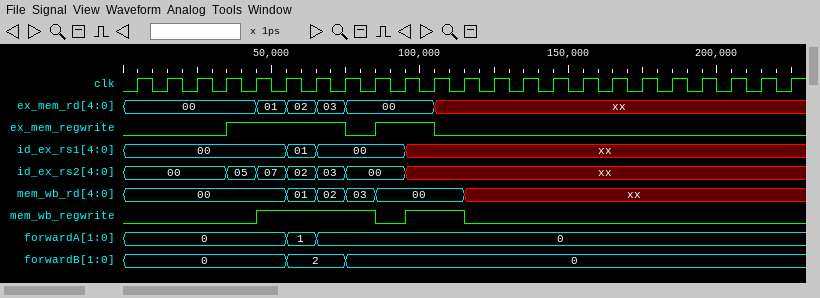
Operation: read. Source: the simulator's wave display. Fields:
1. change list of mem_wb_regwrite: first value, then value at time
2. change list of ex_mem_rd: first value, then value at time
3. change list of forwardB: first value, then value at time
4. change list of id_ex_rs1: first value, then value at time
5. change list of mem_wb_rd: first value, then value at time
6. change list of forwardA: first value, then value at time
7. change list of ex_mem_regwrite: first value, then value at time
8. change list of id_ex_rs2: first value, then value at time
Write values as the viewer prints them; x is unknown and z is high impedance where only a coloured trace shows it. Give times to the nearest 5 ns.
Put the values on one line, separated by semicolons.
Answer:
0, 1 at 45 ns, 0 at 85 ns, 1 at 95 ns, 0 at 115 ns; 00, 01 at 45 ns, 02 at 55 ns, 03 at 65 ns, 00 at 75 ns, xx at 105 ns; 0, 2 at 55 ns, 0 at 75 ns; 00, 01 at 55 ns, 00 at 65 ns, xx at 95 ns; 00, 01 at 55 ns, 02 at 65 ns, 03 at 75 ns, 00 at 85 ns, xx at 115 ns; 0, 1 at 55 ns, 0 at 65 ns; 0, 1 at 35 ns, 0 at 75 ns, 1 at 85 ns, 0 at 105 ns; 00, 05 at 35 ns, 07 at 45 ns, 02 at 55 ns, 03 at 65 ns, 00 at 75 ns, xx at 95 ns
